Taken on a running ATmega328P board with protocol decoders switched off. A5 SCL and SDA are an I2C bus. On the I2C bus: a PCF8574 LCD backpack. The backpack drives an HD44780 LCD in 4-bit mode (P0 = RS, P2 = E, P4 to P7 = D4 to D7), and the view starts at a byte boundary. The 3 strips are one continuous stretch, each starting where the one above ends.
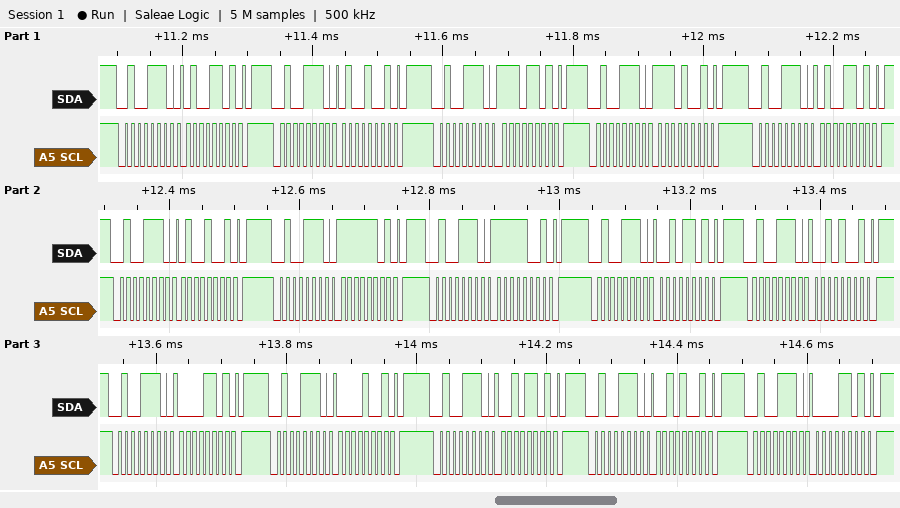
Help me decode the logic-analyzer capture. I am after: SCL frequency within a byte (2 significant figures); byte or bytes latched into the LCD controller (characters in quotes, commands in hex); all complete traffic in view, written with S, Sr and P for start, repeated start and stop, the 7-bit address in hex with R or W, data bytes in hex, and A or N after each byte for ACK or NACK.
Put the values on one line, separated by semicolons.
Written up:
100 kHz; 'N' 'O' ' '; S 27W A 4D A P S 27W A 49 A P S 27W A ED A P S 27W A E9 A P S 27W A 4D A P S 27W A 49 A P S 27W A FD A P S 27W A F9 A P S 27W A 2D A P S 27W A 29 A P S 27W A 0D A P S 27W A 09 A P S 27W A 2D A P S 27W A 29 A P S 27W A 0D A P
